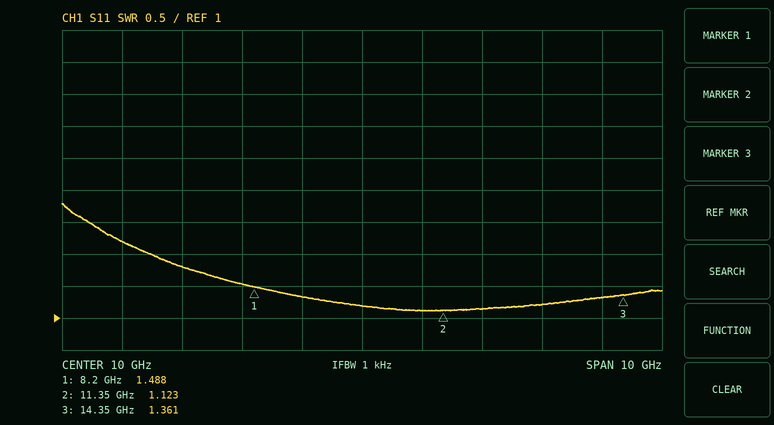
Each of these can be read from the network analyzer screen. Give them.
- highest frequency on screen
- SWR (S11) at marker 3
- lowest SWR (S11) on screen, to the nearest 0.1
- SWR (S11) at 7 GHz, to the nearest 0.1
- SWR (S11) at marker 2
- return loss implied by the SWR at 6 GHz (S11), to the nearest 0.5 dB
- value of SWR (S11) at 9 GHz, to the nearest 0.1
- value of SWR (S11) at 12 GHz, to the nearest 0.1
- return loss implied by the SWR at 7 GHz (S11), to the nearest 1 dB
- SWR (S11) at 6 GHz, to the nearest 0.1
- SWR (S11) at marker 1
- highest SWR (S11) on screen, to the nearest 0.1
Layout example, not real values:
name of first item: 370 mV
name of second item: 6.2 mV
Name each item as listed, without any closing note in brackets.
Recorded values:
highest frequency on screen: 15 GHz
SWR (S11) at marker 3: 1.361
lowest SWR (S11) on screen, to the nearest 0.1: 1.1
SWR (S11) at 7 GHz, to the nearest 0.1: 1.8
SWR (S11) at marker 2: 1.123
return loss implied by the SWR at 6 GHz (S11), to the nearest 0.5 dB: 8.5 dB
value of SWR (S11) at 9 GHz, to the nearest 0.1: 1.3
value of SWR (S11) at 12 GHz, to the nearest 0.1: 1.1
return loss implied by the SWR at 7 GHz (S11), to the nearest 1 dB: 11 dB
SWR (S11) at 6 GHz, to the nearest 0.1: 2.2
SWR (S11) at marker 1: 1.488
highest SWR (S11) on screen, to the nearest 0.1: 2.8
